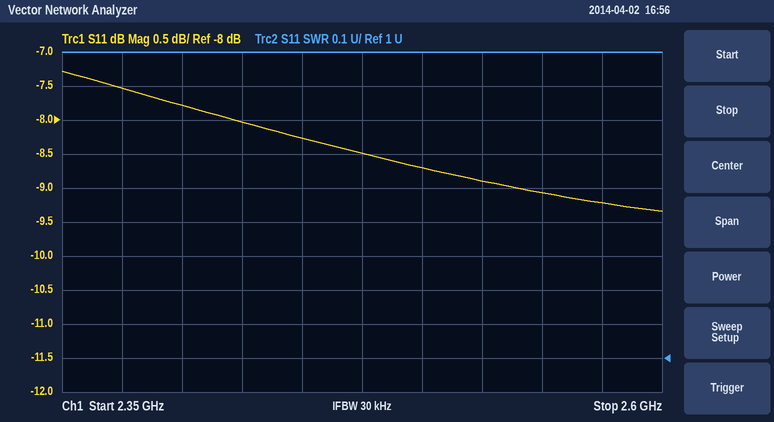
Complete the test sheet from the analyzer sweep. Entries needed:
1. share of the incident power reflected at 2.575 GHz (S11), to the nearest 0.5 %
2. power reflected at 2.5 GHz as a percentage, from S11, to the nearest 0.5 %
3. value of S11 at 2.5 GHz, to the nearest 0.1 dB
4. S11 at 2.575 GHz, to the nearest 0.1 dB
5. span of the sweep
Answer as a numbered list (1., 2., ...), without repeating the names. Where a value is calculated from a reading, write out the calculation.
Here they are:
1. 10^(-9.2/10) ≈ 12.0 %
2. 10^(-8.7/10) ≈ 13.5 %
3. -8.7 dB
4. -9.2 dB
5. 250 MHz
